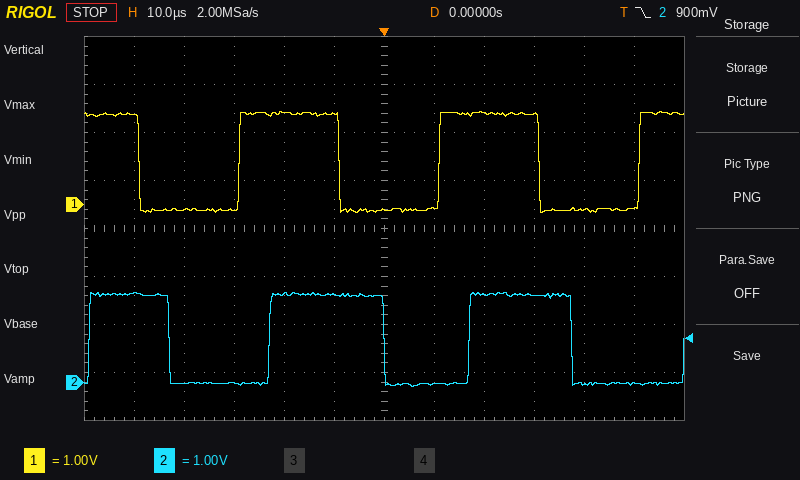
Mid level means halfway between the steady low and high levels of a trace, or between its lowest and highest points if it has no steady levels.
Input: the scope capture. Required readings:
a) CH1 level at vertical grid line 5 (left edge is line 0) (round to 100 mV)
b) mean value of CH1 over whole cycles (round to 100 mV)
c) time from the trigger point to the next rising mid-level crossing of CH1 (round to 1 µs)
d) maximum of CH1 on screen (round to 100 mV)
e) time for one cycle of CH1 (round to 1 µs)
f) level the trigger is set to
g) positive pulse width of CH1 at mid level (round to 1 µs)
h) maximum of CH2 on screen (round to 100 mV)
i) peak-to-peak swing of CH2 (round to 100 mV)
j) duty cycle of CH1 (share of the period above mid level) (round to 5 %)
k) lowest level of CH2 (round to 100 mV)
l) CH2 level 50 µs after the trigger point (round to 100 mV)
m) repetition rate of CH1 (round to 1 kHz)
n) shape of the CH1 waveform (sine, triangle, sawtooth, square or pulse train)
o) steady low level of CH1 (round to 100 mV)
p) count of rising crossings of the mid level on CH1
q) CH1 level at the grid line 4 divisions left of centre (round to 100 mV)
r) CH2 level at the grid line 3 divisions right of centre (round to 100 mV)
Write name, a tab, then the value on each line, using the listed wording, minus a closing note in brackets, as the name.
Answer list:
CH1 level at vertical grid line 5 (left edge is line 0)	1.9 V
mean value of CH1 over whole cycles	900 mV
time from the trigger point to the next rising mid-level crossing of CH1	11 µs
maximum of CH1 on screen	1.9 V
time for one cycle of CH1	40 µs
level the trigger is set to	900 mV
positive pulse width of CH1 at mid level	20 µs
maximum of CH2 on screen	1.9 V
peak-to-peak swing of CH2	2.0 V
duty cycle of CH1 (share of the period above mid level)	50 %
lowest level of CH2	-100 mV
CH2 level 50 µs after the trigger point	0.0 V
repetition rate of CH1	25 kHz
shape of the CH1 waveform	square
steady low level of CH1	-100 mV
count of rising crossings of the mid level on CH1	3
CH1 level at the grid line 4 divisions left of centre	-100 mV
CH2 level at the grid line 3 divisions right of centre	1.8 V
